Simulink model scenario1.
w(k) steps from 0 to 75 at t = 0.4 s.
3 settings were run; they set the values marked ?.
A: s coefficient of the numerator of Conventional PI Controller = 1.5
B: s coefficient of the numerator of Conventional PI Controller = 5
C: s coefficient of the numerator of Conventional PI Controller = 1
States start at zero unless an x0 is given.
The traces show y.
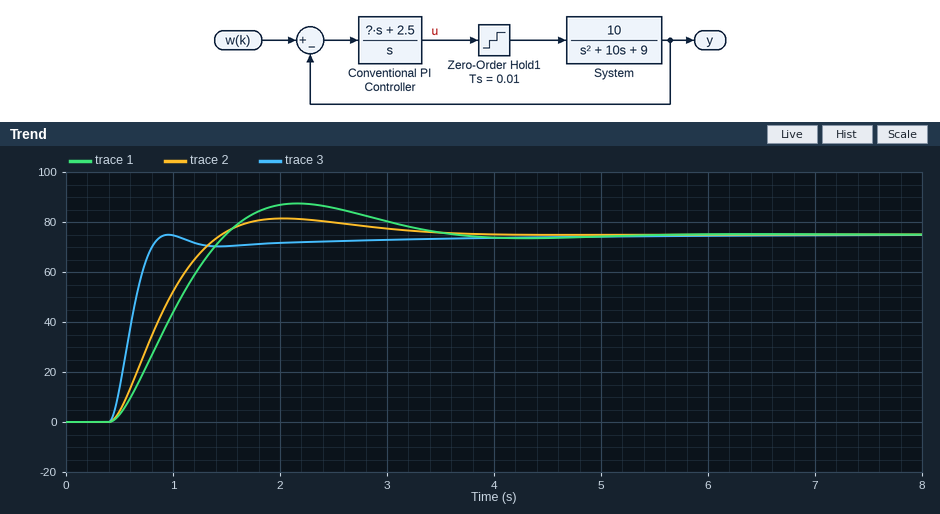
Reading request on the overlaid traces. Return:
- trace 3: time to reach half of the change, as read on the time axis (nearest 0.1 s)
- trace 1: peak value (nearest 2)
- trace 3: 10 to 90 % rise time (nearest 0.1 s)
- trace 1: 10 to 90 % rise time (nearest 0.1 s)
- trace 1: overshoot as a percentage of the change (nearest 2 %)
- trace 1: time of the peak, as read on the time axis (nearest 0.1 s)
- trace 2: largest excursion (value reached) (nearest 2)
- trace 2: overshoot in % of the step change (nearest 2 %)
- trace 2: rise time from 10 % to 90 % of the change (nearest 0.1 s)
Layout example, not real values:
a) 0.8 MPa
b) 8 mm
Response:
a) 0.6 s
b) 88
c) 0.3 s
d) 0.8 s
e) 16 %
f) 2.2 s
g) 82
h) 8 %
i) 0.7 s
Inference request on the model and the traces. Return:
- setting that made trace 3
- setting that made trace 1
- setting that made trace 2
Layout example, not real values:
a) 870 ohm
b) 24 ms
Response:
a) B
b) C
c) A
